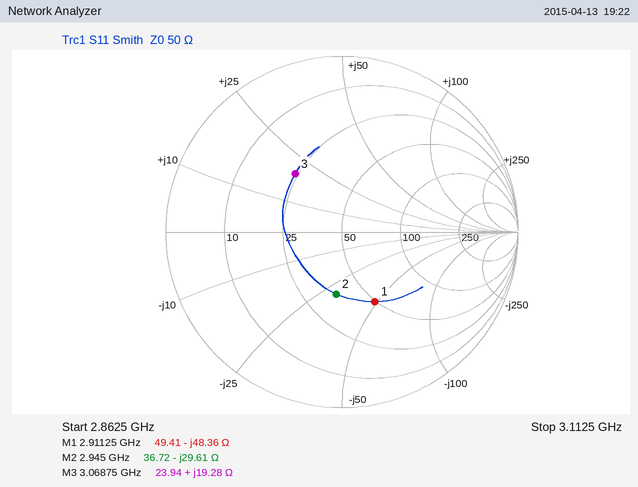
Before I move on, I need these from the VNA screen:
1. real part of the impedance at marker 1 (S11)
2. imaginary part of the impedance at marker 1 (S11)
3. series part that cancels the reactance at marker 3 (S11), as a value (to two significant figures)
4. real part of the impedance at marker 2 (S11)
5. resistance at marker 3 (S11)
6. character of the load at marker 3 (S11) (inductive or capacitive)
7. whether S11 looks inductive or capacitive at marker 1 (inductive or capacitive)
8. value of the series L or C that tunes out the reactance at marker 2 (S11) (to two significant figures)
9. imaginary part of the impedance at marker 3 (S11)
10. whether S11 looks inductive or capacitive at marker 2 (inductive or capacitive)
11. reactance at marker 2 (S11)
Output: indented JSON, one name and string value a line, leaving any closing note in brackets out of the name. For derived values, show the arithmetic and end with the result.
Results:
{
  "real part of the impedance at marker 1": "49.41 Ω",
  "imaginary part of the impedance at marker 1": "-48.36 Ω",
  "series part that cancels the reactance at marker 3 (S11), as a value": "C = 1/(2π × 3.06875 GHz × 19.28 Ω) ≈ 2.7 pF",
  "real part of the impedance at marker 2": "36.72 Ω",
  "resistance at marker 3": "23.94 Ω",
  "character of the load at marker 3 (S11)": "inductive",
  "whether S11 looks inductive or capacitive at marker 1": "capacitive",
  "value of the series L or C that tunes out the reactance at marker 2 (S11)": "L = 29.61 Ω/(2π × 2.945 GHz) ≈ 1.6 nH",
  "imaginary part of the impedance at marker 3": "+19.28 Ω",
  "whether S11 looks inductive or capacitive at marker 2": "capacitive",
  "reactance at marker 2": "-29.61 Ω"
}
